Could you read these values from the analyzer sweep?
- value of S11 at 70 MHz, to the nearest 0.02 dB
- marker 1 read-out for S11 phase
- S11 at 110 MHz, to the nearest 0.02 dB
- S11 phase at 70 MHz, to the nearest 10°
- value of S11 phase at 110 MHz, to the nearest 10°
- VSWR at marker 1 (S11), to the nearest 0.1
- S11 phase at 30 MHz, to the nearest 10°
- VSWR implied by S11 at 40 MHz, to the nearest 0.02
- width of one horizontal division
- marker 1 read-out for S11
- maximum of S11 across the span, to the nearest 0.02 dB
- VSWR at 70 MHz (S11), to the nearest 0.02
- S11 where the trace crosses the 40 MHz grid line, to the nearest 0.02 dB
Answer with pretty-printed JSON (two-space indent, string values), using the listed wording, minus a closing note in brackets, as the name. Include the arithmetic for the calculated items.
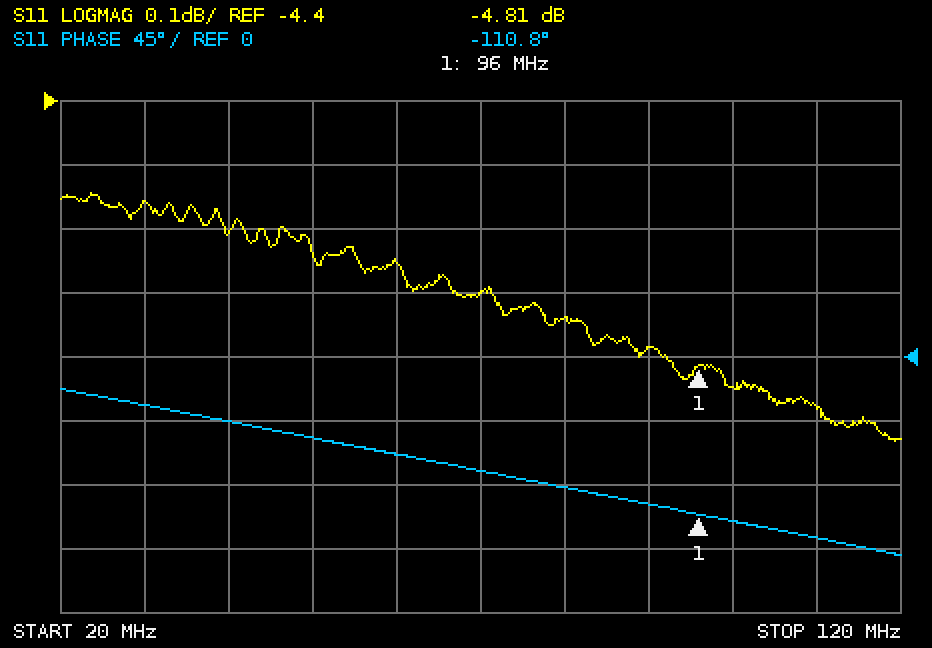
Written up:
{
  "value of S11 at 70 MHz, to the nearest 0.02 dB": "-4.70 dB",
  "marker 1 read-out for S11 phase": "-110.8°",
  "S11 at 110 MHz, to the nearest 0.02 dB": "-4.88 dB",
  "S11 phase at 70 MHz, to the nearest 10°": "-80°",
  "value of S11 phase at 110 MHz, to the nearest 10°": "-130°",
  "VSWR at marker 1 (S11), to the nearest 0.1": "(1 + 0.5748)/(1 − 0.5748) ≈ 3.7",
  "S11 phase at 30 MHz, to the nearest 10°": "-30°",
  "VSWR implied by S11 at 40 MHz, to the nearest 0.02": "|Γ| = 10^(-4.6/20) = 0.5888; VSWR = (1 + 0.5888)/(1 − 0.5888) ≈ 3.86",
  "width of one horizontal division": "10 MHz",
  "marker 1 read-out for S11": "-4.81 dB",
  "maximum of S11 across the span, to the nearest 0.02 dB": "-4.54 dB",
  "VSWR at 70 MHz (S11), to the nearest 0.02": "|Γ| = 10^(-4.7/20) = 0.5821; VSWR = (1 + 0.5821)/(1 − 0.5821) ≈ 3.79, so 3.78 to the nearest 0.02",
  "S11 where the trace crosses the 40 MHz grid line, to the nearest 0.02 dB": "-4.60 dB"
}
